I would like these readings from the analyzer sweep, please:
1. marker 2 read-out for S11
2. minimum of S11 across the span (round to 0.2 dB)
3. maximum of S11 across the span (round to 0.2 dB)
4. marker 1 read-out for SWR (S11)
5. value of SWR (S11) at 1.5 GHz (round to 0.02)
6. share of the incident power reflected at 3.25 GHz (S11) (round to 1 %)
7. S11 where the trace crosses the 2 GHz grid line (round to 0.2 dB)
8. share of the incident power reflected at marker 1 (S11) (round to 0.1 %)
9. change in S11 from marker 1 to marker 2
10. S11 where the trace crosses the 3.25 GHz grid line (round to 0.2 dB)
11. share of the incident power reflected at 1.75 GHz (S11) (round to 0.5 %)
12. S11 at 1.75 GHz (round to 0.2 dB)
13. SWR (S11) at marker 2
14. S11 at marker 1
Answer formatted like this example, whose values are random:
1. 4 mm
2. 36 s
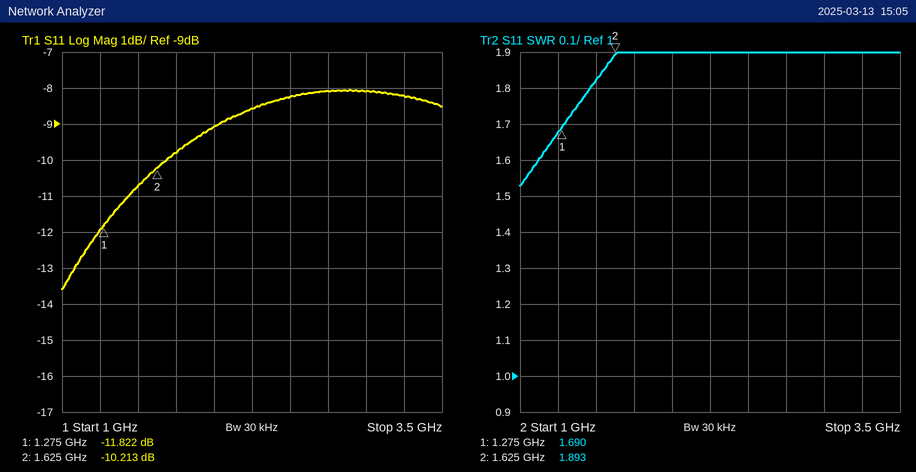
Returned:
1. -10.213 dB
2. -13.6 dB
3. -8.0 dB
4. 1.690
5. 1.82
6. 15 %
7. -9.0 dB
8. 6.6 %
9. 1.609 dB
10. -8.2 dB
11. 10.5 %
12. -9.8 dB
13. 1.893
14. -11.822 dB
